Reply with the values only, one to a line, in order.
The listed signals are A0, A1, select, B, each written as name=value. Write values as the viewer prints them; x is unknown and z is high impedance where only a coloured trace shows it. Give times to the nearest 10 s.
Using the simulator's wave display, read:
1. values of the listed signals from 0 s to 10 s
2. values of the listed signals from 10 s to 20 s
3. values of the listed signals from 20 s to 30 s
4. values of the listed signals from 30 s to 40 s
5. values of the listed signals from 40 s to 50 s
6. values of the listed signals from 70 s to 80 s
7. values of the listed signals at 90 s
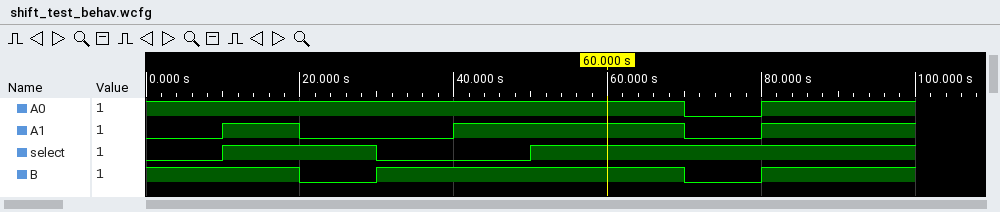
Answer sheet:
A0=1, A1=0, select=0, B=1
A0=1, A1=1, select=1, B=1
A0=1, A1=0, select=1, B=0
A0=1, A1=0, select=0, B=1
A0=1, A1=1, select=0, B=1
A0=0, A1=0, select=1, B=0
A0=1, A1=1, select=1, B=1
